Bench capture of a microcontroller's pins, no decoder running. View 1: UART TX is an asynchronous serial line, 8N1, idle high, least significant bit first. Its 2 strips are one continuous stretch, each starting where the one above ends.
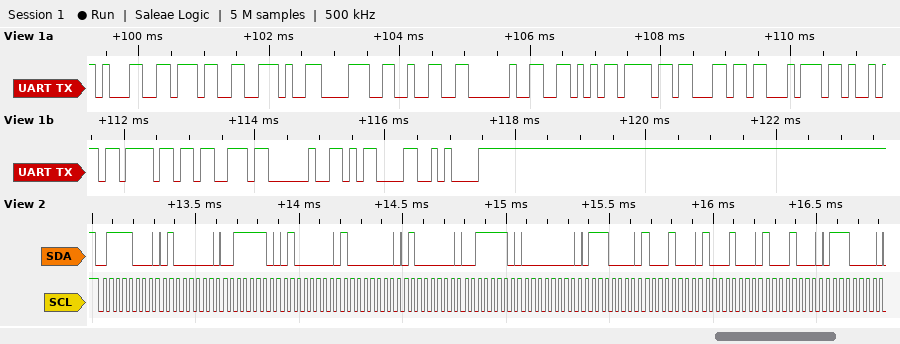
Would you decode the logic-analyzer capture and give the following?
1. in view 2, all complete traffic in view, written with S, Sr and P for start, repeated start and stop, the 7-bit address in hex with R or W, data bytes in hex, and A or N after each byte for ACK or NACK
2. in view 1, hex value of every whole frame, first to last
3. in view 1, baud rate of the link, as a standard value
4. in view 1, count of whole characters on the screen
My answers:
S 3CW A 40 A 3E A 40 A 80 A 40 A 3E A 00 A 70 A 88 A 88 A 88 A 70 A
31 37 2E 38 32 20 56 6F 6C 74 69 6F 73 20 0D 0A
9600 baud
16
